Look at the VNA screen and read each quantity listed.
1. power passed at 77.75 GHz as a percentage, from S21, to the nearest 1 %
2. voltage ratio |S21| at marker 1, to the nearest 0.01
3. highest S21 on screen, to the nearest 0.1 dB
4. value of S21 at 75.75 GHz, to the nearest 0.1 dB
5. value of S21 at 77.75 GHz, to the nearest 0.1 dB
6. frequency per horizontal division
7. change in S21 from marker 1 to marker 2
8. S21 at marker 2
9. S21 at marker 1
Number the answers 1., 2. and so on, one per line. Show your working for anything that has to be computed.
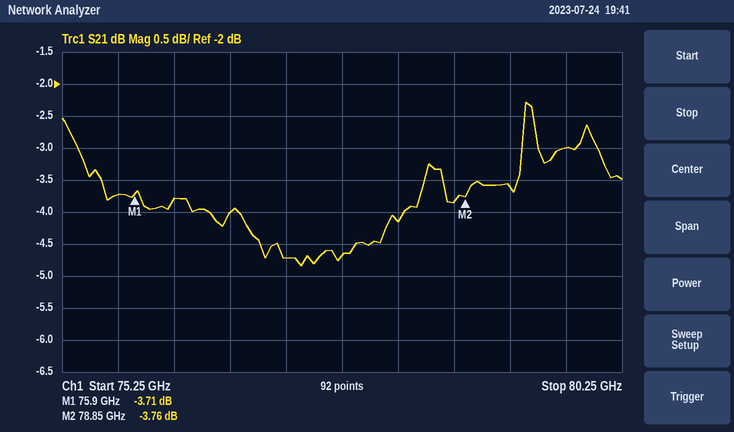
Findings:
1. 10^(-4.7/10) ≈ 34 %
2. 10^(-3.71/20) ≈ 0.65
3. -2.3 dB
4. -3.7 dB
5. -4.7 dB
6. 500 MHz
7. -3.76 − (-3.71) = -0.05 dB
8. -3.76 dB
9. -3.71 dB
